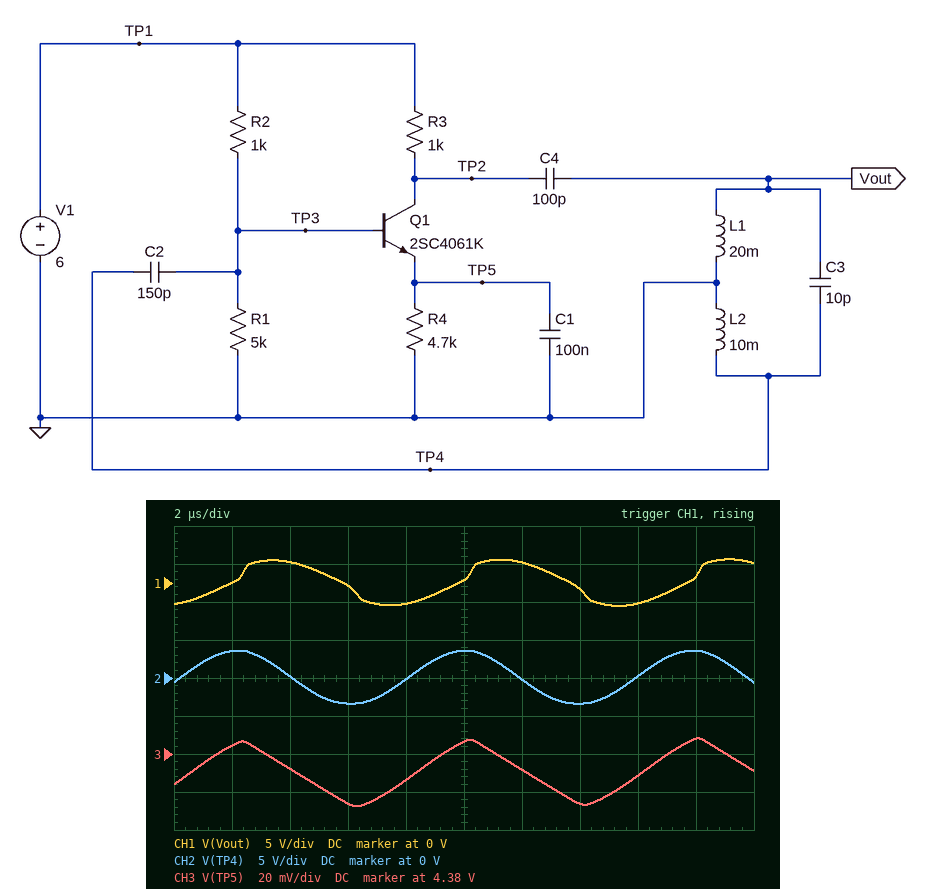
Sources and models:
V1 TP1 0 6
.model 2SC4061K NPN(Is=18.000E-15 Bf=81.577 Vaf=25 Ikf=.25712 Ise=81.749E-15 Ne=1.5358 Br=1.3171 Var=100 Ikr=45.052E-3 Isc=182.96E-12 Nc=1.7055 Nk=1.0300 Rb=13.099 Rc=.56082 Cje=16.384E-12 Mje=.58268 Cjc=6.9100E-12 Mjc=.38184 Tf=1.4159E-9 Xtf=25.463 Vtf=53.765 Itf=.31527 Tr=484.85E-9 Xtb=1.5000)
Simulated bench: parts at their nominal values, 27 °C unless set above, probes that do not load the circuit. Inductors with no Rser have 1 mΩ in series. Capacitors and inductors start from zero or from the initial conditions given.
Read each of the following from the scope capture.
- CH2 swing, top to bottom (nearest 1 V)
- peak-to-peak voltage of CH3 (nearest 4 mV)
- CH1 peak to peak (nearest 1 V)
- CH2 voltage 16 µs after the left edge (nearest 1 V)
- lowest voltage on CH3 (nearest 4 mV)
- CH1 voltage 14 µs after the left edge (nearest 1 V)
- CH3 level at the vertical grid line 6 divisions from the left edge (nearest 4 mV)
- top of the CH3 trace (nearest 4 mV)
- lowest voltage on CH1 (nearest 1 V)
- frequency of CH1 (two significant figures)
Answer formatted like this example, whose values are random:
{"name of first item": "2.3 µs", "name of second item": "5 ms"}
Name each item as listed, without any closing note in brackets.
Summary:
{"CH2 swing, top to bottom": "7 V", "peak-to-peak voltage of CH3": "36 mV", "CH1 peak to peak": "6 V", "CH2 voltage 16 µs after the left edge": "0 V", "lowest voltage on CH3": "4.352 V", "CH1 voltage 14 µs after the left edge": "-1 V", "CH3 level at the vertical grid line 6 divisions from the left edge": "4.372 V", "top of the CH3 trace": "4.388 V", "lowest voltage on CH1": "-3 V", "frequency of CH1": "130 kHz"}
